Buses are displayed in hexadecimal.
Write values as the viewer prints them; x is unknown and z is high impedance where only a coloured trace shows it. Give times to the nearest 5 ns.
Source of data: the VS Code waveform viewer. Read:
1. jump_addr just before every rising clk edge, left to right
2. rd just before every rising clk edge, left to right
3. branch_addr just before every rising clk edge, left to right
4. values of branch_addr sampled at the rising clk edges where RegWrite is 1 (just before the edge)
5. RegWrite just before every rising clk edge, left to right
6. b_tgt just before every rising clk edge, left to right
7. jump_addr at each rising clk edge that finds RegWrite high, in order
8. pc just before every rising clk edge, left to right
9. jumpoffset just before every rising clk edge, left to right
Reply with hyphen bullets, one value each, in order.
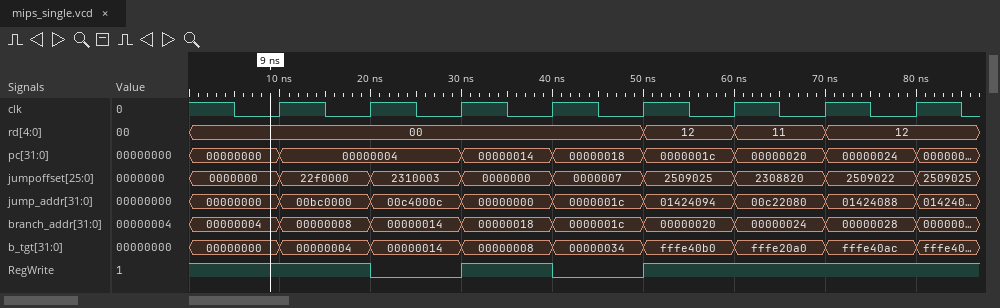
- 00000000, 00bc0000, 00c4000c, 00000000, 0000001c, 01424094, 00c22080, 01424088
- 00, 00, 00, 00, 00, 12, 11, 12
- 00000004, 00000008, 00000014, 00000018, 0000001c, 00000020, 00000024, 00000028
- 00000004, 00000008, 00000018, 00000020, 00000024, 00000028
- 1 1 0 1 0 1 1 1
- 00000000, 00000004, 00000014, 00000008, 00000034, fffe40b0, fffe20a0, fffe40ac
- 00000000, 00bc0000, 00000000, 01424094, 00c22080, 01424088
- 00000000, 00000004, 00000004, 00000014, 00000018, 0000001c, 00000020, 00000024
- 0000000, 22f0000, 2310003, 0000000, 0000007, 2509025, 2308820, 2509022
